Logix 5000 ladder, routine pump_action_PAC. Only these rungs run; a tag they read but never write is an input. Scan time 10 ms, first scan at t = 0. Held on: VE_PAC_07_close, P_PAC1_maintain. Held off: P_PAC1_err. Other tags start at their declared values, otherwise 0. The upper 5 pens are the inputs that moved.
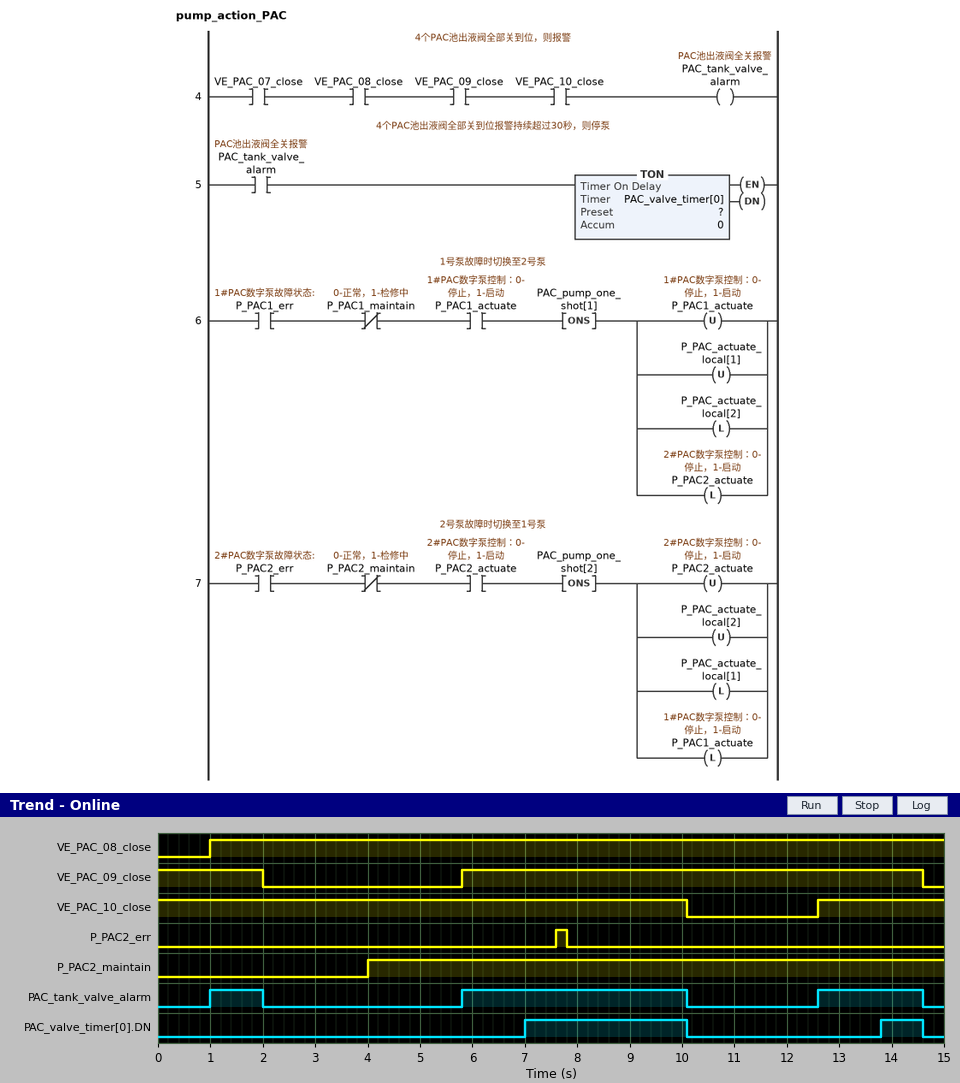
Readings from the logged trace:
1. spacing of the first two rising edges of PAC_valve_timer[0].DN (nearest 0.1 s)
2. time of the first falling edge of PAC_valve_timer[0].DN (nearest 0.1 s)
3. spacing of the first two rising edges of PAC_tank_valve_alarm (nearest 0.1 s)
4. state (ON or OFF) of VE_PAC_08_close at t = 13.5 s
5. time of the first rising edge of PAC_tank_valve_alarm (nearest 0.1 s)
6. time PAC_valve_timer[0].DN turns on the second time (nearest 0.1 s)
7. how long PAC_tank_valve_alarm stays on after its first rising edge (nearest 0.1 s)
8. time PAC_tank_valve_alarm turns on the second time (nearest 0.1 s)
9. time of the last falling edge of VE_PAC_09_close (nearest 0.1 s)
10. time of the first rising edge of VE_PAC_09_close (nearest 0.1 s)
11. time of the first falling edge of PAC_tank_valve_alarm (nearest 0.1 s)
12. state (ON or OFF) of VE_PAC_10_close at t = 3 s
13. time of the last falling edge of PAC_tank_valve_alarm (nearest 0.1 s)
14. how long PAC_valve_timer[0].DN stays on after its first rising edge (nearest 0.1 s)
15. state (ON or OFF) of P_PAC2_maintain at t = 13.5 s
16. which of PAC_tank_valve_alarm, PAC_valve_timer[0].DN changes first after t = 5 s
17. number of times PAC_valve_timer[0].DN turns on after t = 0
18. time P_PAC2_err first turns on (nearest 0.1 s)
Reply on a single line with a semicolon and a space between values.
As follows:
6.8 s; 10.1 s; 4.8 s; ON; 1.0 s; 13.8 s; 1.0 s; 5.8 s; 14.6 s; 5.8 s; 2.0 s; ON; 14.6 s; 3.1 s; ON; PAC_tank_valve_alarm; 2; 7.6 s
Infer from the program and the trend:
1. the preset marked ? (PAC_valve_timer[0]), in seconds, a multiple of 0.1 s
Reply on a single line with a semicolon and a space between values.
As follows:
1.2 s
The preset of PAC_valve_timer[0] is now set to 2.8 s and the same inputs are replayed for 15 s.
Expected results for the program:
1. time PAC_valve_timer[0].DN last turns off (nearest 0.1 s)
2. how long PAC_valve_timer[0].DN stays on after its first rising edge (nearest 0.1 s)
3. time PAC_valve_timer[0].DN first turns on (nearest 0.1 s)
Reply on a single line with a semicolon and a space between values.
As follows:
10.1 s; 1.5 s; 8.6 s
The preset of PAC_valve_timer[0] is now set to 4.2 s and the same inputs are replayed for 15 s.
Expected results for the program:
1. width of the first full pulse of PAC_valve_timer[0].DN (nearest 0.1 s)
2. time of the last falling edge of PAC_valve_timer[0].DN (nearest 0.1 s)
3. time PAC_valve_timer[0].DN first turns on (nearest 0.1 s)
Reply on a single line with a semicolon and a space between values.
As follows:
0.1 s; 10.1 s; 10.0 s
